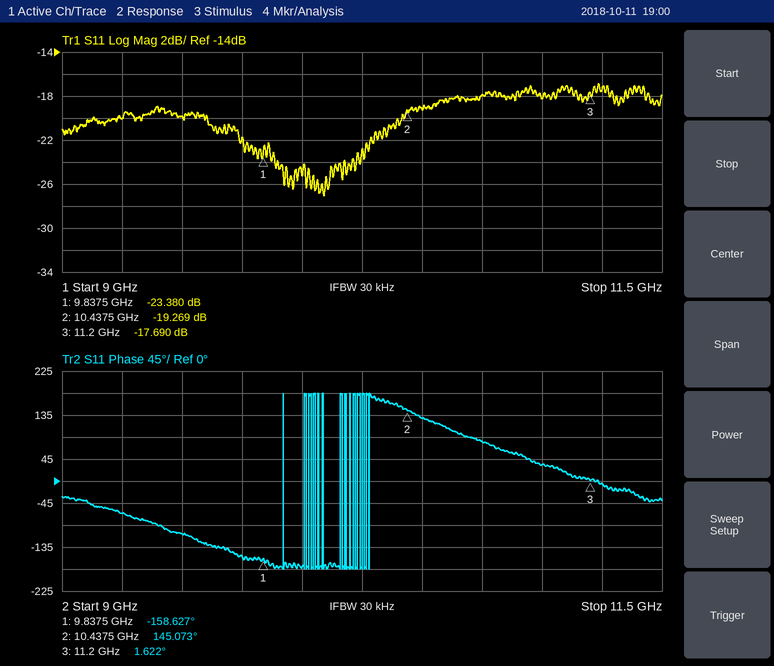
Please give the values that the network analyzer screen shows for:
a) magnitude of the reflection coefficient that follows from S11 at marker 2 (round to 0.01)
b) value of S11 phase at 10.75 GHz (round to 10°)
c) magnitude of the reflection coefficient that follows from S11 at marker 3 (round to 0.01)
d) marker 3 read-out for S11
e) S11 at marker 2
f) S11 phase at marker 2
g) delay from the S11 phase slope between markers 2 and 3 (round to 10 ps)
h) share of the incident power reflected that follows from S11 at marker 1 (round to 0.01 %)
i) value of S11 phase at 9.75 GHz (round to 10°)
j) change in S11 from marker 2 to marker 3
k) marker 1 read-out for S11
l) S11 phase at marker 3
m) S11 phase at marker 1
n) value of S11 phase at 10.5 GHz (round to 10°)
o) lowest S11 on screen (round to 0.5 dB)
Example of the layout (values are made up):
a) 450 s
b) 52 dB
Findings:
a) 0.11
b) 80°
c) 0.13
d) -17.690 dB
e) -19.269 dB
f) 145.073°
g) 520 ps
h) 0.46 %
i) -150°
j) 1.579 dB
k) -23.380 dB
l) 1.622°
m) -158.627°
n) 130°
o) -27.0 dB
